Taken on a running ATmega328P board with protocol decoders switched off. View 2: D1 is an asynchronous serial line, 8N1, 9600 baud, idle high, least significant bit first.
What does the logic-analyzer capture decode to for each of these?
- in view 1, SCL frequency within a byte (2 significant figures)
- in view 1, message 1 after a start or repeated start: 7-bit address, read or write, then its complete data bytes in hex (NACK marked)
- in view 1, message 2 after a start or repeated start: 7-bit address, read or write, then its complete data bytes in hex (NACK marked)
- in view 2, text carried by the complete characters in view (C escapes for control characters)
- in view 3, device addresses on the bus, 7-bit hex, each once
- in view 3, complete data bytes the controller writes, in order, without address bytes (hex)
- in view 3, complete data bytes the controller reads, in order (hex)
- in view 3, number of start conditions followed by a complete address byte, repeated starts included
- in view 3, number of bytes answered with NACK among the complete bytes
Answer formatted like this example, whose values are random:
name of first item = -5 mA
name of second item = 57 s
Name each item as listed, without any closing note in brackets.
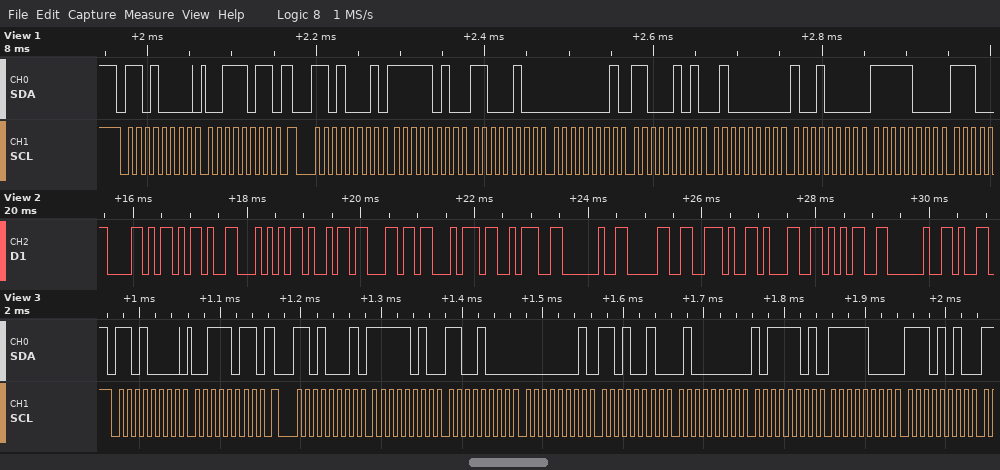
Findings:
in view 1, SCL frequency within a byte = 100 kHz
in view 1, message 1 after a start or repeated start: 7-bit address, read or write, then its complete data bytes in hex = 0x68 write: 3B
in view 1, message 2 after a start or repeated start: 7-bit address, read or write, then its complete data bytes in hex = 0x68 read: FA C4 01 C5 40 90 F8
in view 2, text carried by the complete characters in view = "X-Tilt: 0.15 "
in view 3, device addresses on the bus, 7-bit hex, each once = 0x68
in view 3, complete data bytes the controller writes, in order, without address bytes = 3B
in view 3, complete data bytes the controller reads, in order = FA C8 01 D2 40 BD F8 EA
in view 3, number of start conditions followed by a complete address byte, repeated starts included = 2
in view 3, number of bytes answered with NACK among the complete bytes = 0
